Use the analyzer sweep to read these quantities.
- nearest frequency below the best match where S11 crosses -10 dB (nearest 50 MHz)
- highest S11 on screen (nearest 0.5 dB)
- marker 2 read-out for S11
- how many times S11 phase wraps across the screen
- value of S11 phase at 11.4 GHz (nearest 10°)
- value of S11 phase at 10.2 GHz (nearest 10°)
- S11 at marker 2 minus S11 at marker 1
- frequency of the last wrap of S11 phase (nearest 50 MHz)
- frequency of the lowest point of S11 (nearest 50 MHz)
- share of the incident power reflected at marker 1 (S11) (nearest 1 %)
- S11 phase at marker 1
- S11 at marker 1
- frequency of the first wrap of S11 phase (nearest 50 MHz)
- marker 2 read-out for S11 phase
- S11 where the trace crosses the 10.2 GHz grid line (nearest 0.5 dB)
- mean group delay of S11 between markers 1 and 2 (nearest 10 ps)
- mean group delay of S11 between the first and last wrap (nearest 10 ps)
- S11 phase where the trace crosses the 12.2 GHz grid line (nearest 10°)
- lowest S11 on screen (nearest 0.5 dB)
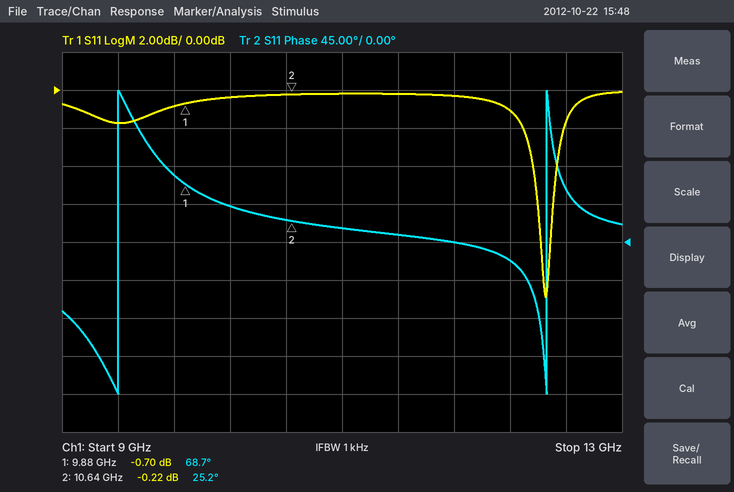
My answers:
12.45 GHz
0.0 dB
-0.22 dB
2
10°
40°
0.48 dB
12.45 GHz
12.45 GHz
85 %
68.7°
-0.70 dB
9.40 GHz
25.2°
-0.5 dB
160 ps
330 ps
-20°
-11.0 dB
